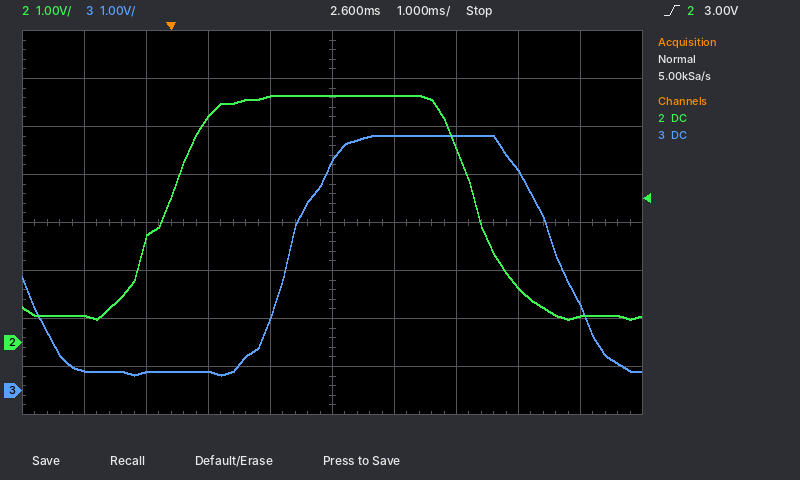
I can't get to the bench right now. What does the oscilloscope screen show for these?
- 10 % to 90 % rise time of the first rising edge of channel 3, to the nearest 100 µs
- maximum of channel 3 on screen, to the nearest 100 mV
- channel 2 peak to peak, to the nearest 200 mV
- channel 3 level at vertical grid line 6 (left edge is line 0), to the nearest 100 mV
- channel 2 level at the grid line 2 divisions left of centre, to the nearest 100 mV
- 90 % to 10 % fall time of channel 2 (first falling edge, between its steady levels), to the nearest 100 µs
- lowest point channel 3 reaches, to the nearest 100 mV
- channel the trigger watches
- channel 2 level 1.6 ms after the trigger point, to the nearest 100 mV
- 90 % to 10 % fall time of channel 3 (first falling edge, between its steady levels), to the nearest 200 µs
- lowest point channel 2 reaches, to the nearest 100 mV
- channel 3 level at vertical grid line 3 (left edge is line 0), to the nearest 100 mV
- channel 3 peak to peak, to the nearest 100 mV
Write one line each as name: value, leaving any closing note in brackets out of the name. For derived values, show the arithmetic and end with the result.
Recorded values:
10 % to 90 % rise time of the first rising edge of channel 3, to the nearest 100 µs: 1.2 ms
maximum of channel 3 on screen, to the nearest 100 mV: 5.3 V
channel 2 peak to peak, to the nearest 200 mV: 4.6 V
channel 3 level at vertical grid line 6 (left edge is line 0), to the nearest 100 mV: 5.3 V
channel 2 level at the grid line 2 divisions left of centre, to the nearest 100 mV: 4.7 V
90 % to 10 % fall time of channel 2 (first falling edge, between its steady levels), to the nearest 100 µs: 1.3 ms
lowest point channel 3 reaches, to the nearest 100 mV: 300 mV
channel the trigger watches: channel 2
channel 2 level 1.6 ms after the trigger point, to the nearest 100 mV: 5.1 V
90 % to 10 % fall time of channel 3 (first falling edge, between its steady levels), to the nearest 200 µs: 1.4 ms
lowest point channel 2 reaches, to the nearest 100 mV: 500 mV
channel 3 level at vertical grid line 3 (left edge is line 0), to the nearest 100 mV: 400 mV
channel 3 peak to peak, to the nearest 100 mV: 5.3 V − (300 mV) = 5.0 V
